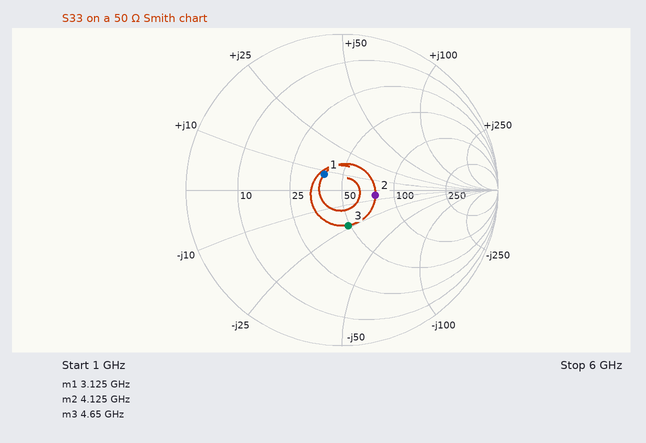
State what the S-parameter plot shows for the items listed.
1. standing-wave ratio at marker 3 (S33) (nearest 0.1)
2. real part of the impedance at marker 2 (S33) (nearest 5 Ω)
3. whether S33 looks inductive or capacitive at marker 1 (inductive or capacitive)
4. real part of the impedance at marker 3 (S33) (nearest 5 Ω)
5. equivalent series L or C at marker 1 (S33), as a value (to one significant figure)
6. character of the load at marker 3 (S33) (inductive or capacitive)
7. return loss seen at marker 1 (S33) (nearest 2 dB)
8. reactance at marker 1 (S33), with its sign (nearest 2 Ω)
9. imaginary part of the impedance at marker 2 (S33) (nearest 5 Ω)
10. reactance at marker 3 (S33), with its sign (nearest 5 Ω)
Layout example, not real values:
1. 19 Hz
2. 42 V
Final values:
1. 1.6
2. 75 Ω
3. inductive
4. 50 Ω
5. 400 pH
6. capacitive
7. 16 dB
8. +8 Ω
9. -5 Ω
10. -25 Ω
